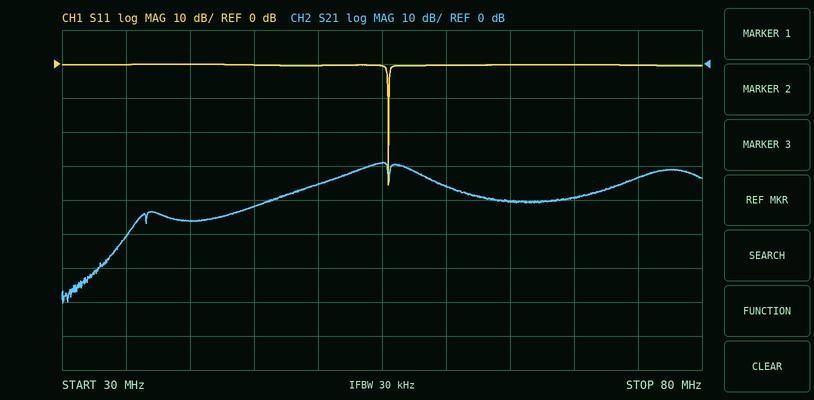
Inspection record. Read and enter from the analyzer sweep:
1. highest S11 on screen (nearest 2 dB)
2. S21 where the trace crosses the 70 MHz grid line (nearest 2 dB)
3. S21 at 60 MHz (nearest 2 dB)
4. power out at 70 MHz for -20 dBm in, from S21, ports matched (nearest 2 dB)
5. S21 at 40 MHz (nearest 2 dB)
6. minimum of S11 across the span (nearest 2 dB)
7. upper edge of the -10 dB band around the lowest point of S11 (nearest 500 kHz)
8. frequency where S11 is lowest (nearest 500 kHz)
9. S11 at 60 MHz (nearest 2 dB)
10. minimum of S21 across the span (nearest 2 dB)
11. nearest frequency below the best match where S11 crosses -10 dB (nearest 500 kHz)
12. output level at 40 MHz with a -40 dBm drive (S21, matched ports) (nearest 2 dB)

0 dB
-40 dB
-36 dB
-60 dBm
-46 dB
-36 dB
55.5 MHz
55.5 MHz
0 dB
-70 dB
55.5 MHz
-86 dBm
